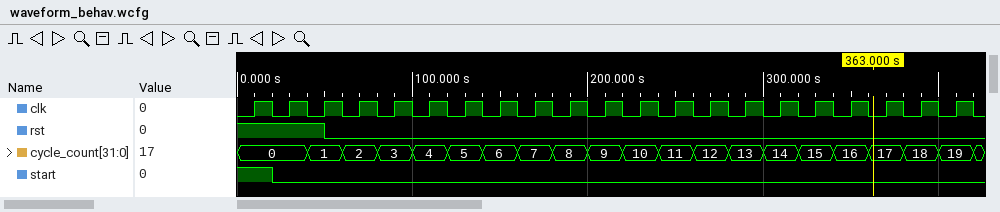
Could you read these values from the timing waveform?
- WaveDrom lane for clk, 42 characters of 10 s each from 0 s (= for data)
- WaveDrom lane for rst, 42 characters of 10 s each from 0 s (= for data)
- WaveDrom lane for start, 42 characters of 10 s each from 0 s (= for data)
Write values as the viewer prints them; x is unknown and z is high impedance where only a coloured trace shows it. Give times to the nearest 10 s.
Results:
{name: 'clk', wave: '010101010101010101010101010101010101010101'}
{name: 'rst', wave: '1....0....................................'}
{name: 'start', wave: '1.0.......................................'}
